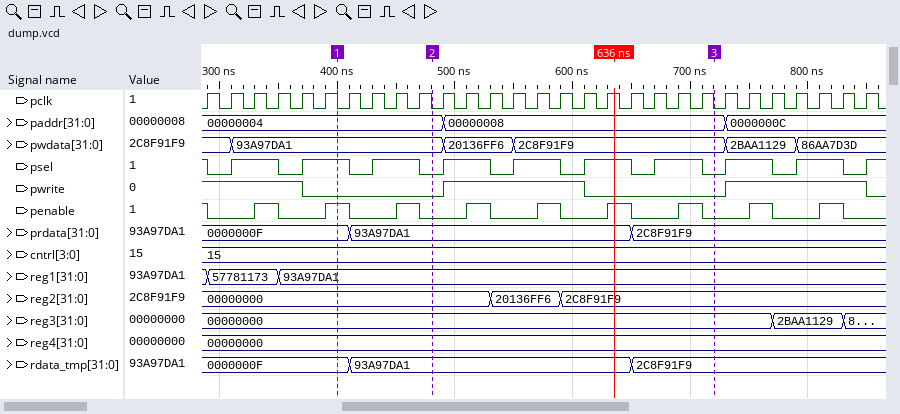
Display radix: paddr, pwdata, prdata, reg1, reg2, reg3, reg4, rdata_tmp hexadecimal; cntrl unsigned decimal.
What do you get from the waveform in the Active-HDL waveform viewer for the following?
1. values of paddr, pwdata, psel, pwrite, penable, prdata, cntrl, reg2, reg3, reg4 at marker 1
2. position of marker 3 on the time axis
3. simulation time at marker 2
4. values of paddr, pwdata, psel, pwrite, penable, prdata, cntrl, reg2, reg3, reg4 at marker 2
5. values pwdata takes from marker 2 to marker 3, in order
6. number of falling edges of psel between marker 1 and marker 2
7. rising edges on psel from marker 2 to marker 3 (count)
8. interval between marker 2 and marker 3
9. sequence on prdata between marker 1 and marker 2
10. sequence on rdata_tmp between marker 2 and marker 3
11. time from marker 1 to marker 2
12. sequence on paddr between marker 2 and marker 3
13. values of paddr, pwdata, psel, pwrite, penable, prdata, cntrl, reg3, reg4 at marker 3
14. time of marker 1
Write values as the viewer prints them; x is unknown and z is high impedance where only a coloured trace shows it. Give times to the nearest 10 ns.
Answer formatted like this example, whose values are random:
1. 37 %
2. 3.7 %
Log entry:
1. paddr=00000004, pwdata=93A97DA1, psel=1, pwrite=0, penable=1, prdata=0000000F, cntrl=15, reg2=00000000, reg3=00000000, reg4=00000000
2. 720 ns
3. 480 ns
4. paddr=00000004, pwdata=93A97DA1, psel=0, pwrite=0, penable=0, prdata=93A97DA1, cntrl=15, reg2=00000000, reg3=00000000, reg4=00000000
5. 93A97DA1, 20136FF6, 2C8F91F9
6. 2
7. 4
8. 240 ns
9. 0000000F, 93A97DA1
10. 93A97DA1, 2C8F91F9
11. 80 ns
12. 00000004, 00000008
13. paddr=00000008, pwdata=2C8F91F9, psel=0, pwrite=0, penable=0, prdata=2C8F91F9, cntrl=15, reg3=00000000, reg4=00000000
14. 400 ns
